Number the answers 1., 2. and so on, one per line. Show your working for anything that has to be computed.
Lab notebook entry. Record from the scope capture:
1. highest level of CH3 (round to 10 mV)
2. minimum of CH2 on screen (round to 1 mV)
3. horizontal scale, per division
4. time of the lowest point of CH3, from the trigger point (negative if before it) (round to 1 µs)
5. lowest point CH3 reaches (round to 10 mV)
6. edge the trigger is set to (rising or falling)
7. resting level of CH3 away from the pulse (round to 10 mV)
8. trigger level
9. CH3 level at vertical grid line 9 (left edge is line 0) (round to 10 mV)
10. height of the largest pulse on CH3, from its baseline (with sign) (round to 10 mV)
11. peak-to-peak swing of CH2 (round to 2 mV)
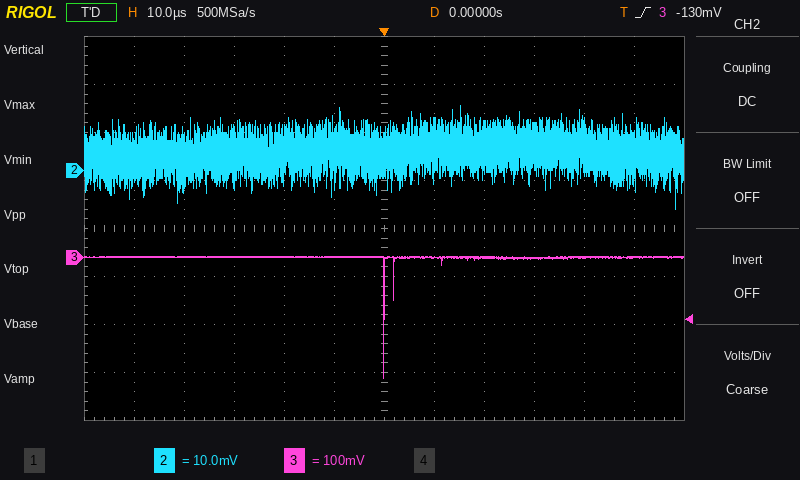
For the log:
1. 0 mV
2. -8 mV
3. 10 µs
4. 0 µs
5. -250 mV
6. rising
7. 0 mV
8. -130 mV
9. 0 mV
10. -250 mV − (0 mV) = -250 mV
11. 22 mV
